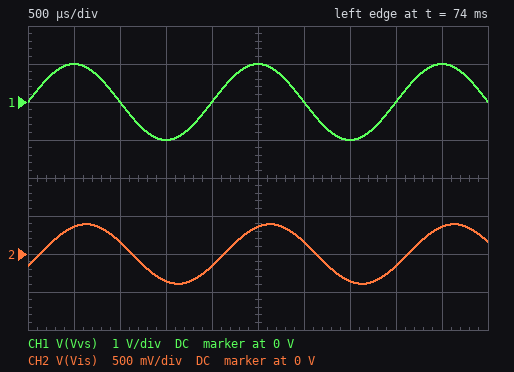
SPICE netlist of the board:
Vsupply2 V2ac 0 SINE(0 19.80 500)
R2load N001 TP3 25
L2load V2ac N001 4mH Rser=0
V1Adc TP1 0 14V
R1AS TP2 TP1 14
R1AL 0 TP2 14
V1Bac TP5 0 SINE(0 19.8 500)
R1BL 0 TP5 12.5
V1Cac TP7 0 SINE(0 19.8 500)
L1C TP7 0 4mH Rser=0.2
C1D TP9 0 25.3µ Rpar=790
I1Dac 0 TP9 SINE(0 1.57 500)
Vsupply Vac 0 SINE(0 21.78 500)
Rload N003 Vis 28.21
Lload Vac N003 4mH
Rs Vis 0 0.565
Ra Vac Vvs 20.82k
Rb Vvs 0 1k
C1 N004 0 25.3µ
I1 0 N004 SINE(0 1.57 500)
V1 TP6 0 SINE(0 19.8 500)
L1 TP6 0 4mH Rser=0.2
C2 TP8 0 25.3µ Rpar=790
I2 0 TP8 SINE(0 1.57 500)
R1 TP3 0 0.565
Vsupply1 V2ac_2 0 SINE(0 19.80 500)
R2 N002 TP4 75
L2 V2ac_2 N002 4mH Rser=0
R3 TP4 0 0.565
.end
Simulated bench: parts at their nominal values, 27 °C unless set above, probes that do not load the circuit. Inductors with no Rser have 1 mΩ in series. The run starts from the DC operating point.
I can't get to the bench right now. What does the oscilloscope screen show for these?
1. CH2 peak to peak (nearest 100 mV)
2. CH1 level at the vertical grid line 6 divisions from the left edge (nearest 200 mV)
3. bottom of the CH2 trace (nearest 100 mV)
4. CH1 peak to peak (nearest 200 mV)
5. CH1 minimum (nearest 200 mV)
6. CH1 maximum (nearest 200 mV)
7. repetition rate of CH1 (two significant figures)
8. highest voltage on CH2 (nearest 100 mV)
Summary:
800 mV
0 V
-400 mV
2.0 V
-1.0 V
1.0 V
500 Hz
400 mV
